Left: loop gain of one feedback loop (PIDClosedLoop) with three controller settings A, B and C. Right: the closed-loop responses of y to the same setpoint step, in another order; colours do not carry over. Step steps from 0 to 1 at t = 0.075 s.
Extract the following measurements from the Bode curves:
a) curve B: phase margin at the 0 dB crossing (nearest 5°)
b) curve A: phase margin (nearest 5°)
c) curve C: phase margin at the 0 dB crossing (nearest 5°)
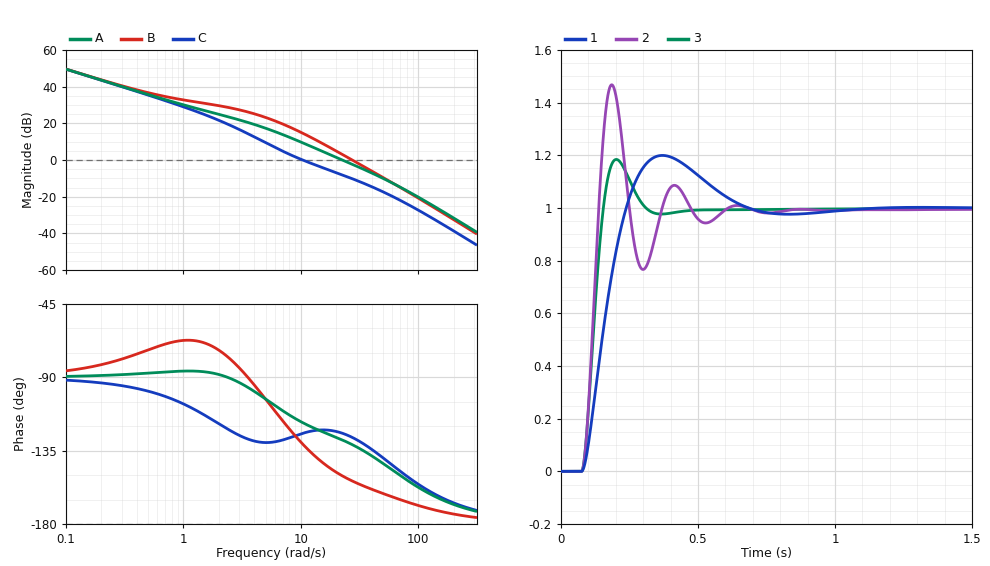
25°
50°
55°
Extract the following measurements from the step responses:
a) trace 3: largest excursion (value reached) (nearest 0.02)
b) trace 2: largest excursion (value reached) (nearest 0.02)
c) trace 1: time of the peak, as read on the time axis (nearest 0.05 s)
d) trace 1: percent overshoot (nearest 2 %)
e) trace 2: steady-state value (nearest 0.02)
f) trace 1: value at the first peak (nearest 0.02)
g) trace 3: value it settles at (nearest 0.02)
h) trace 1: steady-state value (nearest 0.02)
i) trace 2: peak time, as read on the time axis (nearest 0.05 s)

1.18
1.46
0.35 s
20 %
1.00
1.20
1.00
1.00
0.20 s
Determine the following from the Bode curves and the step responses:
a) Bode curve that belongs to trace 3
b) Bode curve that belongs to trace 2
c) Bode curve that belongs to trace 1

A
B
C
